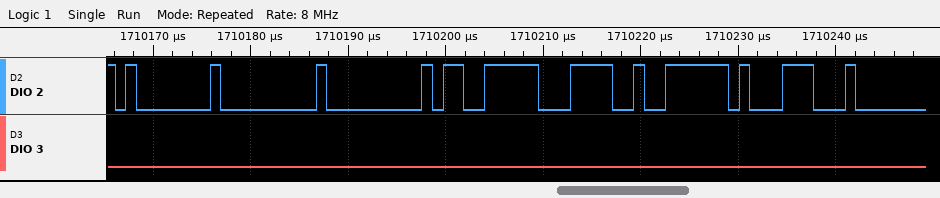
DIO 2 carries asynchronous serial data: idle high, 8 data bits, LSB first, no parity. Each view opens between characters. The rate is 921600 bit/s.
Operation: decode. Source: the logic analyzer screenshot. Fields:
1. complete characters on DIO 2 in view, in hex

01, 00, 00, F3, 3C, 7E, 1C
